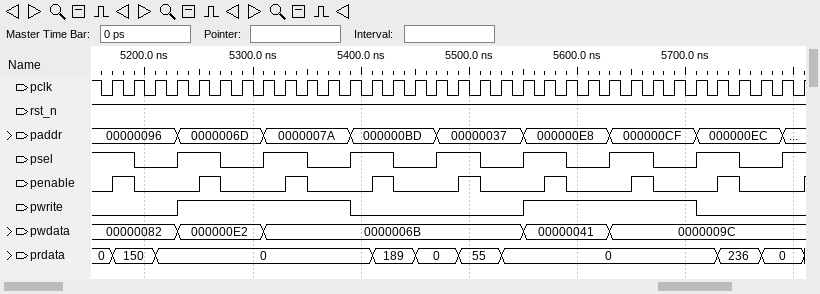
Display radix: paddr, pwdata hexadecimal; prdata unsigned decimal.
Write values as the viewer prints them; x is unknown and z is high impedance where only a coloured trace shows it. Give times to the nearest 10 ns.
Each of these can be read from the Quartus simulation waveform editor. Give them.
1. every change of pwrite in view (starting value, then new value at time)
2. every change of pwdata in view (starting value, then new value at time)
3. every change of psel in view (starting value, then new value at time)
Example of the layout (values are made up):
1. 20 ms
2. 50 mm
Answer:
1. 0, 1 at 5230 ns, 0 at 5390 ns, 1 at 5550 ns, 0 at 5710 ns
2. 00000082, 000000E2 at 5230 ns, 0000006B at 5310 ns, 00000041 at 5550 ns, 0000009C at 5630 ns
3. 1, 0 at 5190 ns, 1 at 5230 ns, 0 at 5270 ns, 1 at 5310 ns, 0 at 5350 ns, 1 at 5390 ns, 0 at 5430 ns, 1 at 5470 ns, 0 at 5510 ns, 1 at 5550 ns, 0 at 5590 ns, 1 at 5630 ns, 0 at 5670 ns, 1 at 5710 ns, 0 at 5750 ns, 1 at 5790 ns
